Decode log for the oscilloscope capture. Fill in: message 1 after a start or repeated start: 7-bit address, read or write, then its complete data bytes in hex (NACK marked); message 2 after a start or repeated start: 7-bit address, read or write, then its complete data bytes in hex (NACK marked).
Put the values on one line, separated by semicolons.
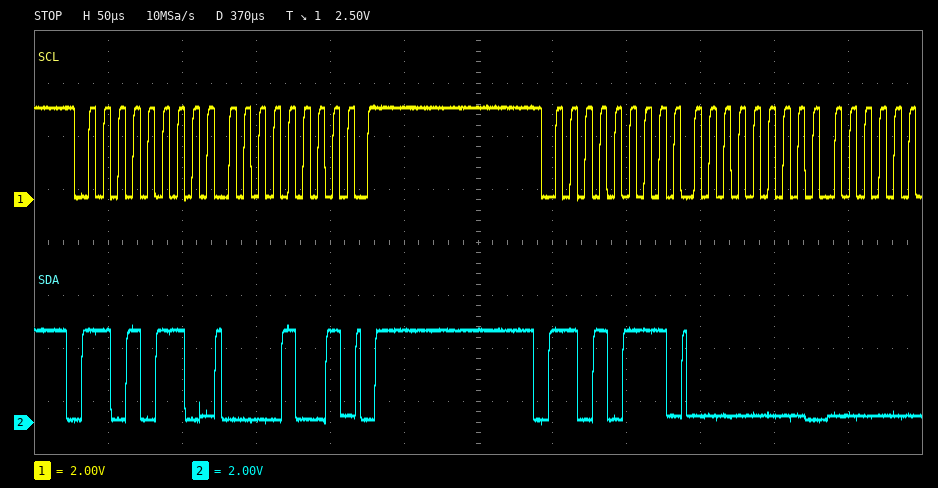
0x6B write: 09; 0x6B read: 00
